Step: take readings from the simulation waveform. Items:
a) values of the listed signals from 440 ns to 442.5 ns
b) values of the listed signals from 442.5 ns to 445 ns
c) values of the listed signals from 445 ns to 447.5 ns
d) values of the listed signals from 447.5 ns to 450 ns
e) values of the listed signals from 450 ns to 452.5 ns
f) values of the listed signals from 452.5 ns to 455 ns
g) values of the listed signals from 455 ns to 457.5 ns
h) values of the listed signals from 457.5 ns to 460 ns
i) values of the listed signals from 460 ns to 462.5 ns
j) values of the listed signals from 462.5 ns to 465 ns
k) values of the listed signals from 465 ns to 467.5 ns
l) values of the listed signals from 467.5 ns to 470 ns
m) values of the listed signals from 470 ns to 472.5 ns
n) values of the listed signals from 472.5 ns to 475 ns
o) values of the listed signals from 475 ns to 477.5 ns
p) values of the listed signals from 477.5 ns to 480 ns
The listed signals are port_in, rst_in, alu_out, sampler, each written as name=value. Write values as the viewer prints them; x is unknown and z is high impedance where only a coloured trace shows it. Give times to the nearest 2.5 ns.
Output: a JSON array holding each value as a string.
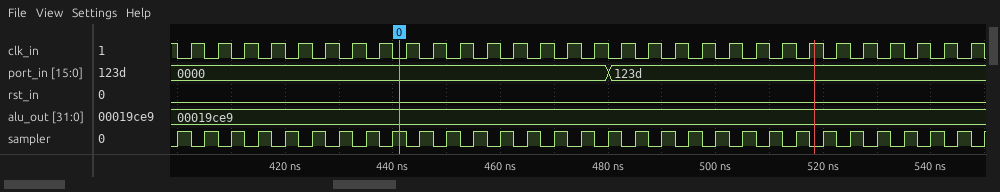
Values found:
["port_in=0000, rst_in=0, alu_out=00019ce9, sampler=1", "port_in=0000, rst_in=0, alu_out=00019ce9, sampler=0", "port_in=0000, rst_in=0, alu_out=00019ce9, sampler=1", "port_in=0000, rst_in=0, alu_out=00019ce9, sampler=0", "port_in=0000, rst_in=0, alu_out=00019ce9, sampler=1", "port_in=0000, rst_in=0, alu_out=00019ce9, sampler=0", "port_in=0000, rst_in=0, alu_out=00019ce9, sampler=1", "port_in=0000, rst_in=0, alu_out=00019ce9, sampler=0", "port_in=0000, rst_in=0, alu_out=00019ce9, sampler=1", "port_in=0000, rst_in=0, alu_out=00019ce9, sampler=0", "port_in=0000, rst_in=0, alu_out=00019ce9, sampler=1", "port_in=0000, rst_in=0, alu_out=00019ce9, sampler=0", "port_in=0000, rst_in=0, alu_out=00019ce9, sampler=1", "port_in=0000, rst_in=0, alu_out=00019ce9, sampler=0", "port_in=0000, rst_in=0, alu_out=00019ce9, sampler=1", "port_in=0000, rst_in=0, alu_out=00019ce9, sampler=0"]
